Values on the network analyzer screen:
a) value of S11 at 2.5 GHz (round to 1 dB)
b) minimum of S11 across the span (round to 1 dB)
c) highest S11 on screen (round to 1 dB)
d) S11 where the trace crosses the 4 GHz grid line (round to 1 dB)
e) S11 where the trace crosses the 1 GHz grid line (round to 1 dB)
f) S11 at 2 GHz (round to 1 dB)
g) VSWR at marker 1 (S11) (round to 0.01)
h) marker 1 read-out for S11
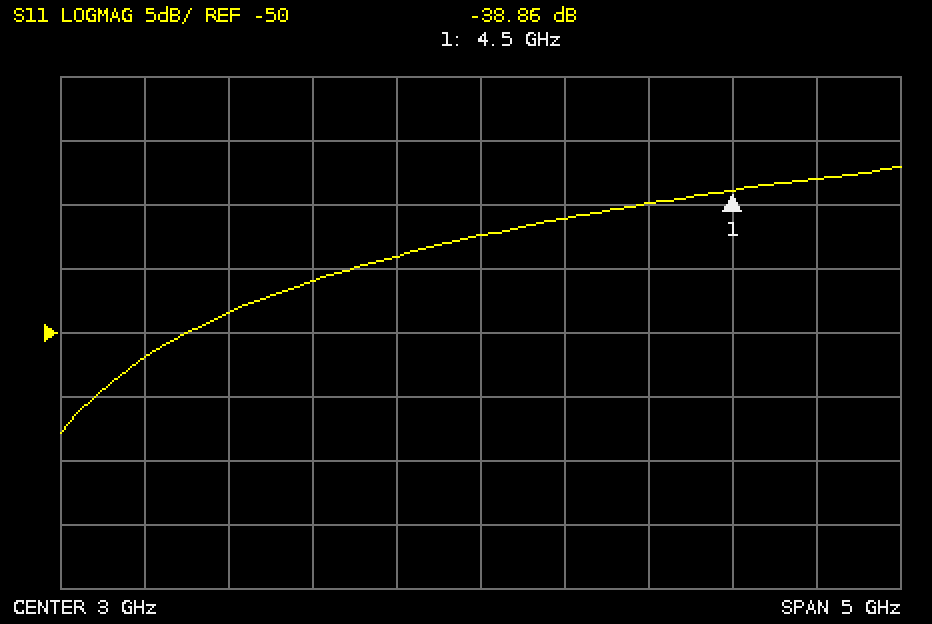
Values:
-44 dB
-58 dB
-37 dB
-40 dB
-52 dB
-46 dB
1.02
-38.86 dB
